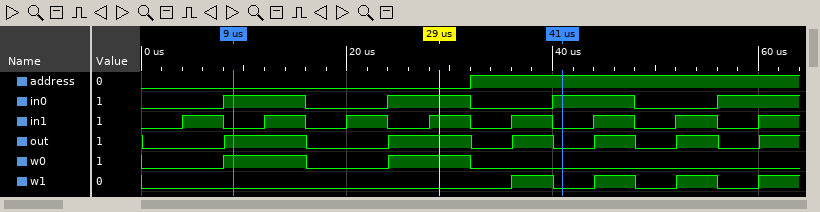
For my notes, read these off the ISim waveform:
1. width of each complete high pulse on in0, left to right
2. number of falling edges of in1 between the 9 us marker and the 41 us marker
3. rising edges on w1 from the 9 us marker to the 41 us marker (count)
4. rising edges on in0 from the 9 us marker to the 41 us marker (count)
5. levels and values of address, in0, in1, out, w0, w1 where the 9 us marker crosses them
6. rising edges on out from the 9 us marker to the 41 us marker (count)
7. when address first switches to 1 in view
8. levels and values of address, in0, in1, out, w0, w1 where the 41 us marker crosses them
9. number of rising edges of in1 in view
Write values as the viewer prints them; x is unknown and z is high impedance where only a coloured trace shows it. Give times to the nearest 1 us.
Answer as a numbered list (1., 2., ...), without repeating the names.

1. 8 us, 8 us, 8 us
2. 4
3. 1
4. 2
5. address=0, in0=1, in1=0, out=1, w0=1, w1=0
6. 2
7. 32 us
8. address=1, in0=1, in1=0, out=0, w0=0, w1=0
9. 8
